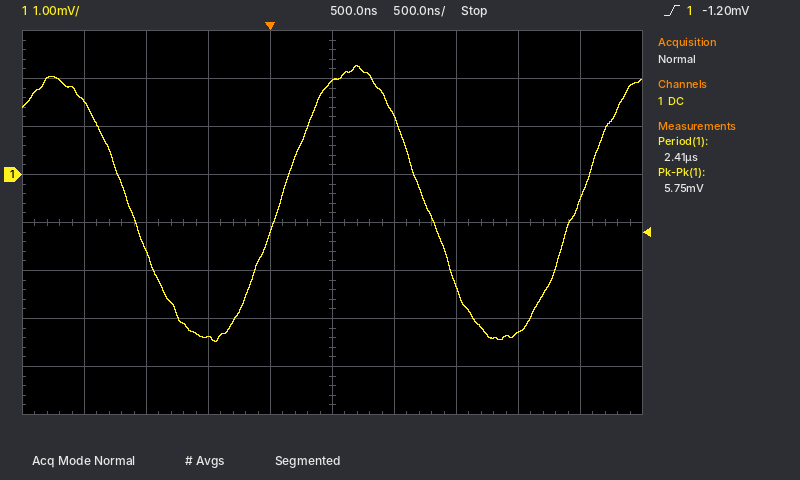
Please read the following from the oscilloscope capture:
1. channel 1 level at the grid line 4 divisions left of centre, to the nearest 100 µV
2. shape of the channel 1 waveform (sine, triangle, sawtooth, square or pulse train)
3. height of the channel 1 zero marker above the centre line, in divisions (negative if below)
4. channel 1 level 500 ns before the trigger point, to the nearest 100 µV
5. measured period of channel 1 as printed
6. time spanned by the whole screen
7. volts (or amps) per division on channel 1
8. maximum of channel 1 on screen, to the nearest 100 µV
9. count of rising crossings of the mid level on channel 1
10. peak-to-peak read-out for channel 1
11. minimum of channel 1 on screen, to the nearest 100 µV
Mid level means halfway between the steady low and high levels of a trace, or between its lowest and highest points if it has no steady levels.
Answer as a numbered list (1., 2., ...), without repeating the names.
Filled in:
1. 1.5 mV
2. sine
3. +1.0 div
4. -3.4 mV
5. 2.41 µs
6. 5 µs
7. 1 mV
8. 2.3 mV
9. 2
10. 5.75 mV
11. -3.5 mV
